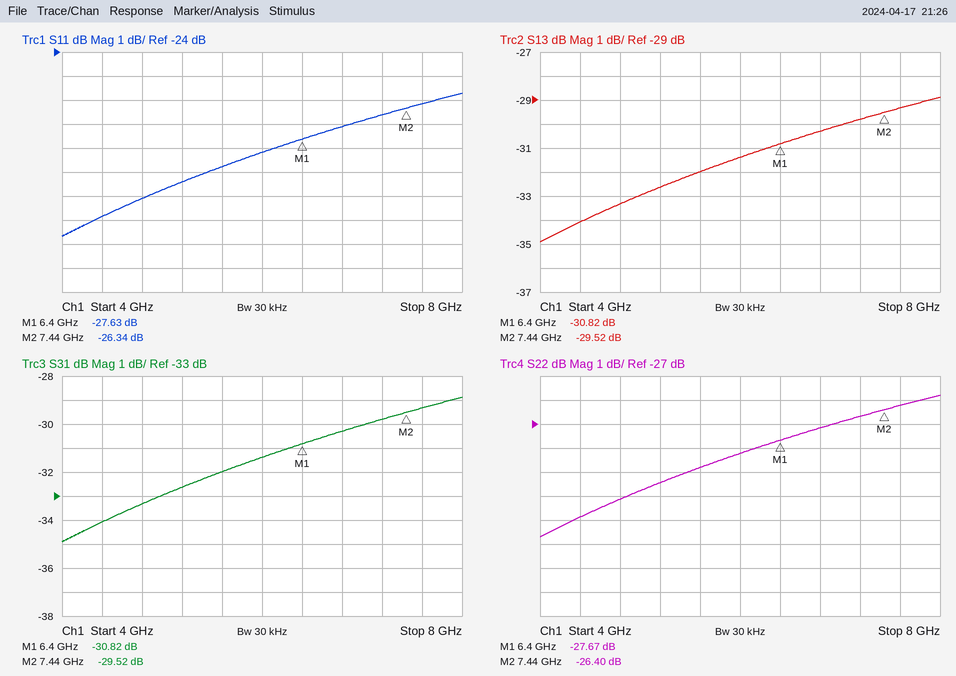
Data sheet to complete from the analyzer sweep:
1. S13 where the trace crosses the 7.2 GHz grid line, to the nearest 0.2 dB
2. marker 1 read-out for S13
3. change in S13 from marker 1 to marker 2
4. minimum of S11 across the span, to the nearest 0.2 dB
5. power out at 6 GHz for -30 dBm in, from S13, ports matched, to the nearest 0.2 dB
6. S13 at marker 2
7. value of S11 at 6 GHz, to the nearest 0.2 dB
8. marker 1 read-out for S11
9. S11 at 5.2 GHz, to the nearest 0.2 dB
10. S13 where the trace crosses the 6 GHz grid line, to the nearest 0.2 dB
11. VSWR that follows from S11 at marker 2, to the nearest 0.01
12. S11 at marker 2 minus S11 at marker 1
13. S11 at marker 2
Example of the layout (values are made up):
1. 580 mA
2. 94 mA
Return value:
1. -29.8 dB
2. -30.82 dB
3. 1.30 dB
4. -31.6 dB
5. -61.4 dBm
6. -29.52 dB
7. -28.2 dB
8. -27.63 dB
9. -29.4 dB
10. -31.4 dB
11. 1.10
12. 1.29 dB
13. -26.34 dB
